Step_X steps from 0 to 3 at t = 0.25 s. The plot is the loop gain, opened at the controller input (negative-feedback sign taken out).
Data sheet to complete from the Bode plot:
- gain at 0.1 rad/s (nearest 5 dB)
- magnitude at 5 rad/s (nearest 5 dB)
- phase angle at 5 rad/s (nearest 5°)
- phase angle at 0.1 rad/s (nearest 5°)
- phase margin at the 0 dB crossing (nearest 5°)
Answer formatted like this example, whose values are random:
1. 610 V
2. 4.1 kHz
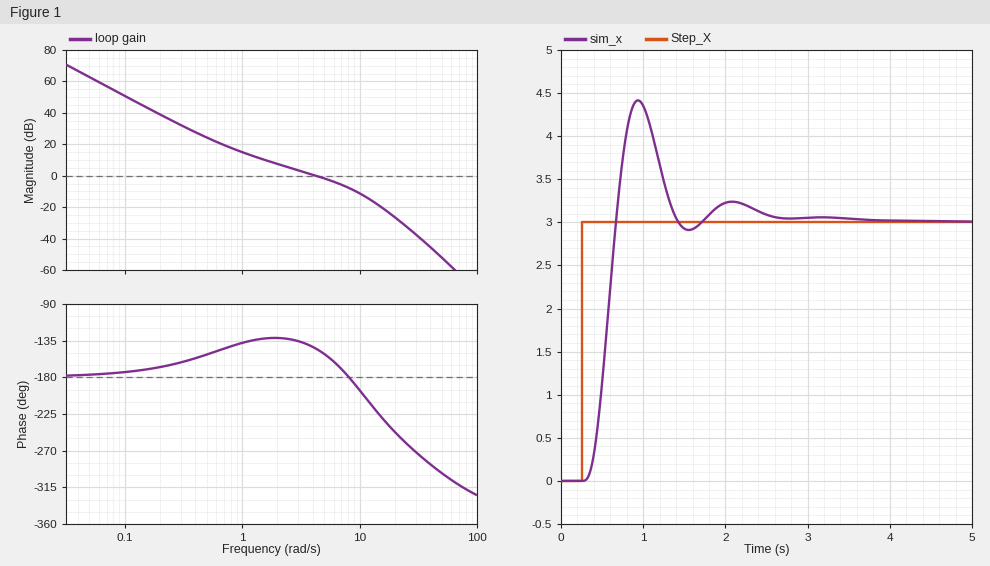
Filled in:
1. 50 dB
2. 0 dB
3. -150°
4. -175°
5. 35°
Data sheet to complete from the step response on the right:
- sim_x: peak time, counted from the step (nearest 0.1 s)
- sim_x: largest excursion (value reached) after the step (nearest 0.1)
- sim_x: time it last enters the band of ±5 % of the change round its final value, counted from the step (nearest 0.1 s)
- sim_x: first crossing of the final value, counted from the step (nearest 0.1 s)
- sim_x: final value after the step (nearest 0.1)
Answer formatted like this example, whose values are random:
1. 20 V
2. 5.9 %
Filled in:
1. 0.7 s
2. 4.4
3. 2.1 s
4. 0.4 s
5. 3.0
